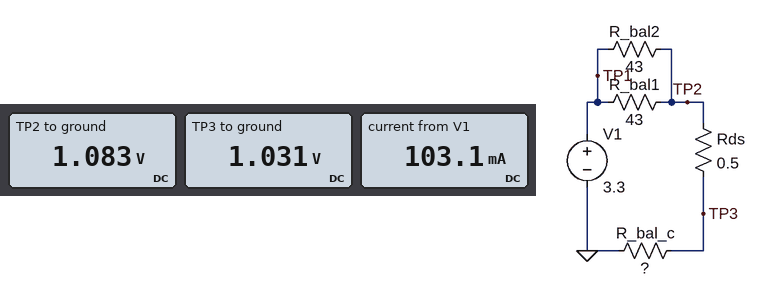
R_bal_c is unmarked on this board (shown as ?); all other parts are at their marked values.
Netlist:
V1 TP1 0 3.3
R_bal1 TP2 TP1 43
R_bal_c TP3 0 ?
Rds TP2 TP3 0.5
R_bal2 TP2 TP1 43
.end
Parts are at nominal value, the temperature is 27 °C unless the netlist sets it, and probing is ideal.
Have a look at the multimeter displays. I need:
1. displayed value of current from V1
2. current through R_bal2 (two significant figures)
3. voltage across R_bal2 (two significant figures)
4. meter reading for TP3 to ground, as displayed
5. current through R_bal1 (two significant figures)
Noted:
103.1 mA
52 mA
2.2 V
1.031 V
52 mA
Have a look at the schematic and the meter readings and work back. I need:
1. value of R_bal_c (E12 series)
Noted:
10 Ω
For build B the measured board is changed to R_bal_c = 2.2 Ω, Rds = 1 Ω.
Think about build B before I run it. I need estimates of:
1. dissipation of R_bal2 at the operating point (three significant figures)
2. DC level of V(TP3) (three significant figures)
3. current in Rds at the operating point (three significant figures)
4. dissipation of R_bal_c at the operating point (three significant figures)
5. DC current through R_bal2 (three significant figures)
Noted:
192 mW
294 mV
134 mA
39.3 mW
66.8 mA
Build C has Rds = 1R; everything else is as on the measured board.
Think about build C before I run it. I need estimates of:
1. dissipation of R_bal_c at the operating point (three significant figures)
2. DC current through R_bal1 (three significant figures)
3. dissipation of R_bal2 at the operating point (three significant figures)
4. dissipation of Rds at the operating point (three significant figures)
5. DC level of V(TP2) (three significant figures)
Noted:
103 mW
50.8 mA
111 mW
10.3 mW
1.12 V
